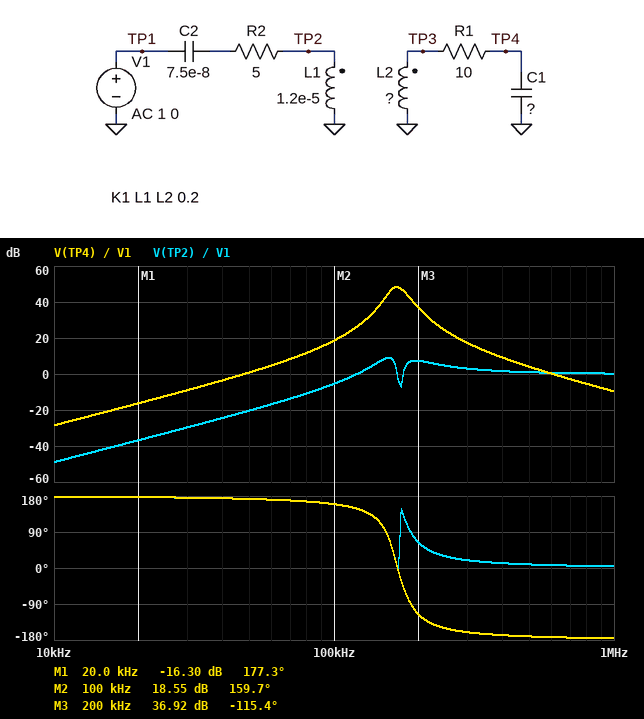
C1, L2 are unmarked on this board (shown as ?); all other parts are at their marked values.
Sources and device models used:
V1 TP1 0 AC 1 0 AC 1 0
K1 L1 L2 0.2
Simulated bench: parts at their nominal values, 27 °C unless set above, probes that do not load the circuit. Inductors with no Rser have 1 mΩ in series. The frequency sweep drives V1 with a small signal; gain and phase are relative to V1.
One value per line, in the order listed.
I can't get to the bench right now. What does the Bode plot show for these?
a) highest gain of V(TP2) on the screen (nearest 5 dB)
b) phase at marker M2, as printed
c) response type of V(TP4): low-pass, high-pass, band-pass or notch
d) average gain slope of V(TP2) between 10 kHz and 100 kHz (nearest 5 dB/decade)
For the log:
10 dB
159.7 deg
band-pass
45 dB/decade
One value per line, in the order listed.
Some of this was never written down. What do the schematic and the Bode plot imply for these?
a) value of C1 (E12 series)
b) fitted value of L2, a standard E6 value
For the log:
27 pF
33 mH
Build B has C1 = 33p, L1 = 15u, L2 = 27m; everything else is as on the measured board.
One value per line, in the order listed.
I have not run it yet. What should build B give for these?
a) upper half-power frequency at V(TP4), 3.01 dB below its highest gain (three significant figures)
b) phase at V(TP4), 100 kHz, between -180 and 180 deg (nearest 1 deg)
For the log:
181 kHz
157 deg
